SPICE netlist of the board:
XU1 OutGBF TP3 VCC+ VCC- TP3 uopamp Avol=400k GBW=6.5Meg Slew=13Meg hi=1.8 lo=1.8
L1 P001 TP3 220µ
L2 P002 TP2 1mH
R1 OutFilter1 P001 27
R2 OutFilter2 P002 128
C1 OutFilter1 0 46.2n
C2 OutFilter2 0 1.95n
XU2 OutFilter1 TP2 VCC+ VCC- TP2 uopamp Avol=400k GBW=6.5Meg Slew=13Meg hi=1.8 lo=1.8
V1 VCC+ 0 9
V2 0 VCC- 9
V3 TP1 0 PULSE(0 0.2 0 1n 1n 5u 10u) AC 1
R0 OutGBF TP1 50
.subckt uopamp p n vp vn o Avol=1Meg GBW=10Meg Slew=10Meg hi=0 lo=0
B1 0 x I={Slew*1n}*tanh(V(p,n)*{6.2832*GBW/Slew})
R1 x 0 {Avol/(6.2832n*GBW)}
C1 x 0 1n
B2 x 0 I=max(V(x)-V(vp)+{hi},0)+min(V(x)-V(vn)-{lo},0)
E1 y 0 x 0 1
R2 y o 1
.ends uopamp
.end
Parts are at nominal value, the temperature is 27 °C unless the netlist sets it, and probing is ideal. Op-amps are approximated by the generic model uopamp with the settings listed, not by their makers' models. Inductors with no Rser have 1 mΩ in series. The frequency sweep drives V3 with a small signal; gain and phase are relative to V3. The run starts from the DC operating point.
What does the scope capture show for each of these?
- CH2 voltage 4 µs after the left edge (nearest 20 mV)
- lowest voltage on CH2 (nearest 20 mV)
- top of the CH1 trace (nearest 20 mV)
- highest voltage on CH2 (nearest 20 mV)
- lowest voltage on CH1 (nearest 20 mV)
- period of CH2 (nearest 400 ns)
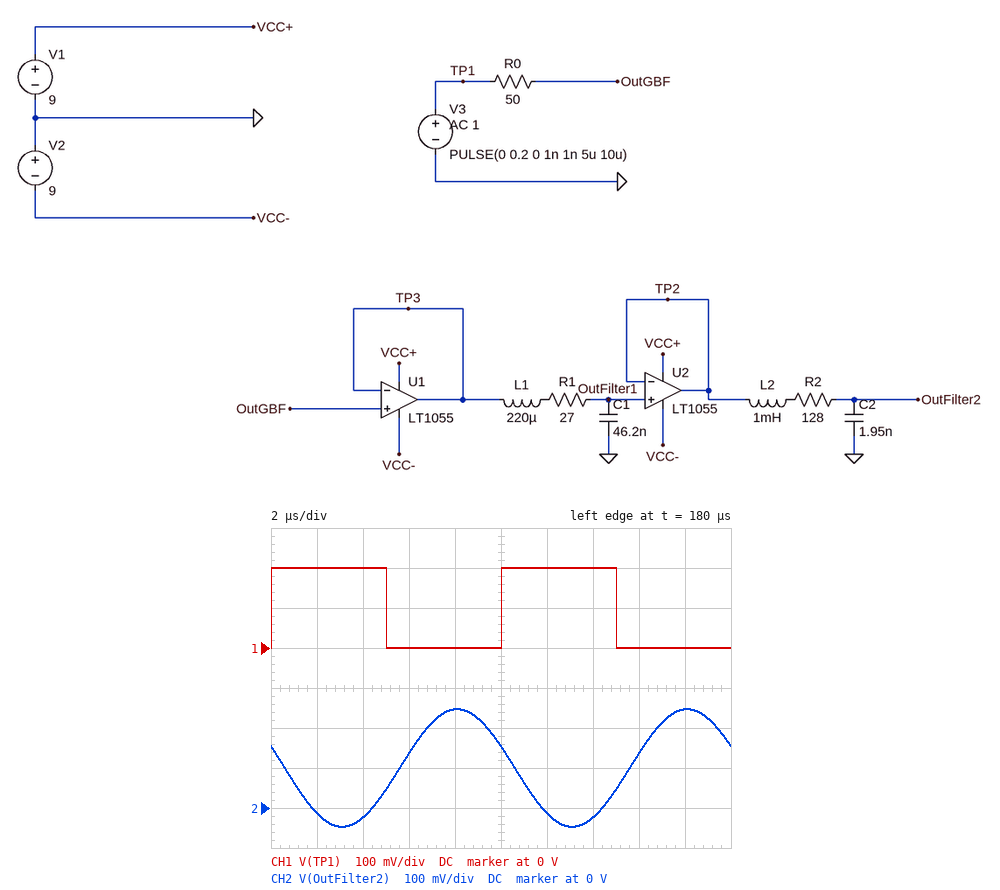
-20 mV
-40 mV
200 mV
240 mV
0 V
10.0 µs
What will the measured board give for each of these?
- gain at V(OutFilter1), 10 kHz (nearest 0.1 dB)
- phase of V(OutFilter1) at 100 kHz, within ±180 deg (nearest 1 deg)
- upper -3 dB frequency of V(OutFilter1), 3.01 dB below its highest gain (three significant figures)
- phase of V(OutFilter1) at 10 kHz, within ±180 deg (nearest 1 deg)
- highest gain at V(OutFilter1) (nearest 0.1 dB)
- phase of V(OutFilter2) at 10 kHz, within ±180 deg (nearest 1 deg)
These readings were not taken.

0.3 dB
-166 deg
57.1 kHz
-5 deg
8.3 dB
-6 deg
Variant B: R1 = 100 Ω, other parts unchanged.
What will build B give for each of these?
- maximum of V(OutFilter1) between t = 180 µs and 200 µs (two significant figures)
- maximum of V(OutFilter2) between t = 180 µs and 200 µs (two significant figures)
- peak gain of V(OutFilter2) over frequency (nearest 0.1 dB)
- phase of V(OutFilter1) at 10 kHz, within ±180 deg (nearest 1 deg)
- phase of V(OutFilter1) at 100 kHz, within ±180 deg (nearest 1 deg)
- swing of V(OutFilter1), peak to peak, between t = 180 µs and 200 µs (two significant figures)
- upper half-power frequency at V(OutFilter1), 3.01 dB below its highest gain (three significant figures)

130 mV
210 mV
0.7 dB
-17 deg
-137 deg
62 mV
48.7 kHz
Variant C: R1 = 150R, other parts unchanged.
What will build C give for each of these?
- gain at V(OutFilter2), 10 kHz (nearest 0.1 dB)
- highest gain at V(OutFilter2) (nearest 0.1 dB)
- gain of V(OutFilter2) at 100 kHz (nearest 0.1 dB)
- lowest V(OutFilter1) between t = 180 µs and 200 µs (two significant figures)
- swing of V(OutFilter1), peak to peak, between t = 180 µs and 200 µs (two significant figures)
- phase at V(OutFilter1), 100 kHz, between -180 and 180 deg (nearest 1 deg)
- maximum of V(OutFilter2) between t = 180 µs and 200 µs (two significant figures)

-0.4 dB
0 dB
-3.4 dB
75 mV
50 mV
-126 deg
190 mV
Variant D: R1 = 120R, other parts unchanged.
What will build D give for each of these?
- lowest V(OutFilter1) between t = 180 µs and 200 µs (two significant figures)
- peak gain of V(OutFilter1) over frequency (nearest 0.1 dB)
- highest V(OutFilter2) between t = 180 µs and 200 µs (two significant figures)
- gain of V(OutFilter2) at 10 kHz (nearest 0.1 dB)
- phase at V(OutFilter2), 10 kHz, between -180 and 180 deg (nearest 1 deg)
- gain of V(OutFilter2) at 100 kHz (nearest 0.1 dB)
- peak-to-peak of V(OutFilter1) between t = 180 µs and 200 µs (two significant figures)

72 mV
0 dB
200 mV
-0.1 dB
-21 deg
-2.2 dB
57 mV
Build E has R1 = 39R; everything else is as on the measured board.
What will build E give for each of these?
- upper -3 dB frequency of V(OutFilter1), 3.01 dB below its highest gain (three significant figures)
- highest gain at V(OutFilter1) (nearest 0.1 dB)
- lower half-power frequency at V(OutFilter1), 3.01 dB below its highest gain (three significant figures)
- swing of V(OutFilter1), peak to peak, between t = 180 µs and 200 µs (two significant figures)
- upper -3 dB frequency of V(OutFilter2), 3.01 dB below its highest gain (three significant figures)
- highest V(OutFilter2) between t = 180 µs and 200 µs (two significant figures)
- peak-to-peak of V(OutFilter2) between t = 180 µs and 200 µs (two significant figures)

58.7 kHz
5.3 dB
27.3 kHz
78 mV
62.5 kHz
240 mV
280 mV
